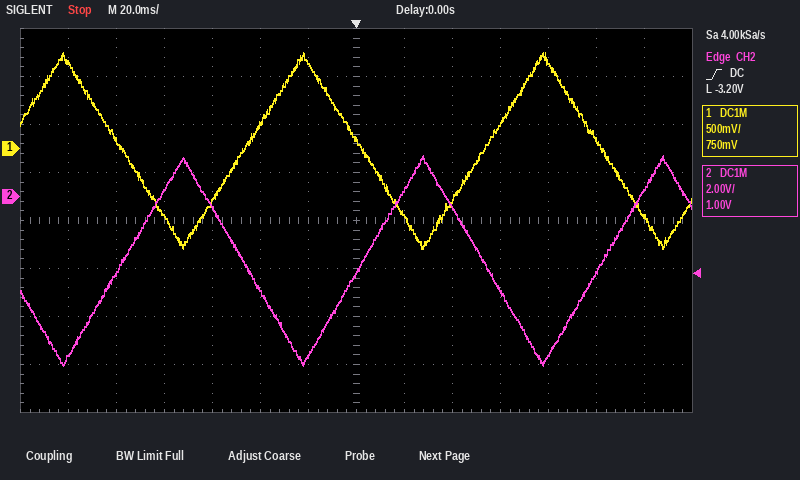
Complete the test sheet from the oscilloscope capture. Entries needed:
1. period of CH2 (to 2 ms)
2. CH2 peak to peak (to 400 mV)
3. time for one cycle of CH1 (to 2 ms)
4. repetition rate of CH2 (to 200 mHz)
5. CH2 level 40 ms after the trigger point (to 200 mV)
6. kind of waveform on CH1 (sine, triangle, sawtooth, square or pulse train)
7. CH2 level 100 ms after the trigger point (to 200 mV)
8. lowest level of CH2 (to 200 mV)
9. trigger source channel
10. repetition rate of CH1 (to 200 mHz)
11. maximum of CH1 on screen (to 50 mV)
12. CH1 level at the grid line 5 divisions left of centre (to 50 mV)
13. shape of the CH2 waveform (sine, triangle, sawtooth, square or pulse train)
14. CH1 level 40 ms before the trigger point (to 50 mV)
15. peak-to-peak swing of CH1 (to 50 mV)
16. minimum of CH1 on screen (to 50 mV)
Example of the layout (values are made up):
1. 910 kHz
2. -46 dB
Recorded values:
1. 100 ms
2. 8.8 V
3. 100 ms
4. 10.0 Hz
5. -400 mV
6. triangle
7. -3.2 V
8. -7.0 V
9. CH2
10. 10.0 Hz
11. 1.00 V
12. 100 mV
13. triangle
14. 250 mV
15. 2.05 V
16. -1.05 V
